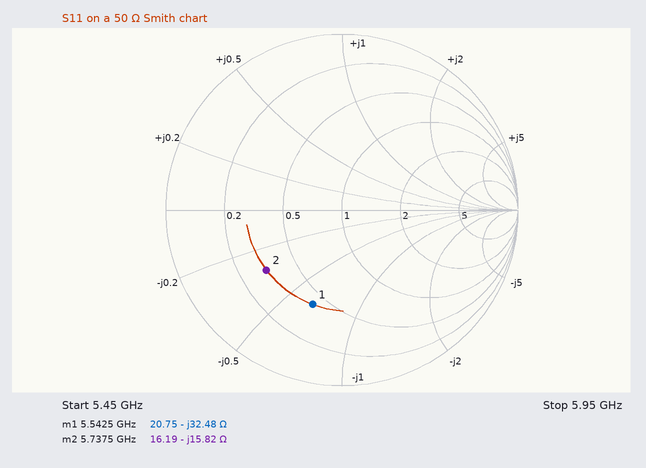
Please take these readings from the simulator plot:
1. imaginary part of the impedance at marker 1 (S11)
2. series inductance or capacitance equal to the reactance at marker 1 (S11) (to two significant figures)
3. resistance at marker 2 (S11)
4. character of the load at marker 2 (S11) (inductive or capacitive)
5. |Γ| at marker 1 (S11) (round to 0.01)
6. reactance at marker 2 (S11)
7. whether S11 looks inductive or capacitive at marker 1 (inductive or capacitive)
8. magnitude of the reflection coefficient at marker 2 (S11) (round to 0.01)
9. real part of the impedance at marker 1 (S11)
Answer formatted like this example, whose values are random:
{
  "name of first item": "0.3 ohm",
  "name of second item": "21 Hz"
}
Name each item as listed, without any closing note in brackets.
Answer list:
{
  "imaginary part of the impedance at marker 1": "-32.48 Ω",
  "series inductance or capacitance equal to the reactance at marker 1 (S11)": "880 fF",
  "resistance at marker 2": "16.19 Ω",
  "character of the load at marker 2 (S11)": "capacitive",
  "|Γ| at marker 1 (S11)": "0.56",
  "reactance at marker 2": "-15.82 Ω",
  "whether S11 looks inductive or capacitive at marker 1": "capacitive",
  "magnitude of the reflection coefficient at marker 2 (S11)": "0.55",
  "real part of the impedance at marker 1": "20.75 Ω"
}
